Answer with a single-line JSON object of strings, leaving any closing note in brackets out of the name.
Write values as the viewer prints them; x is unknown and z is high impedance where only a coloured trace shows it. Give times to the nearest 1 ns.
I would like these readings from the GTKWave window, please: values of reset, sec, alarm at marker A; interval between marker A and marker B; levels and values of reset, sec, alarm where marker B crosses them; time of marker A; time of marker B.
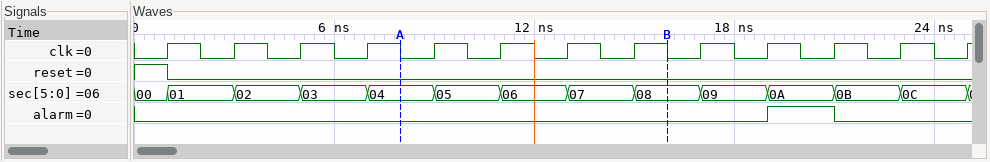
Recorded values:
{"values of reset, sec, alarm at marker A": "reset=0, sec=04, alarm=0", "interval between marker A and marker B": "8 ns", "levels and values of reset, sec, alarm where marker B crosses them": "reset=0, sec=08, alarm=0", "time of marker A": "8 ns", "time of marker B": "16 ns"}
